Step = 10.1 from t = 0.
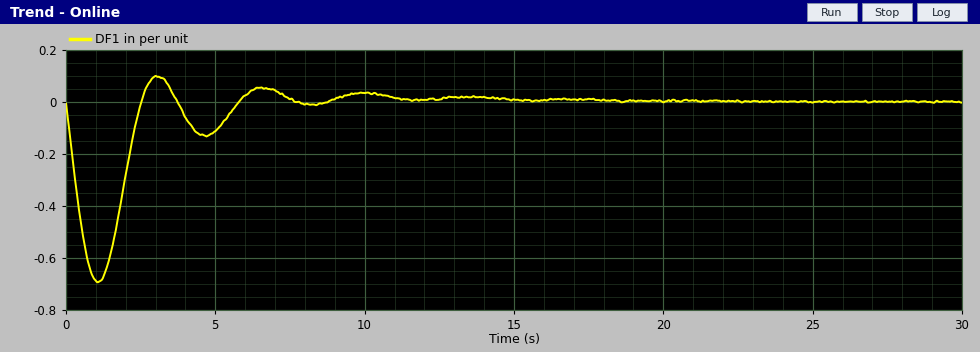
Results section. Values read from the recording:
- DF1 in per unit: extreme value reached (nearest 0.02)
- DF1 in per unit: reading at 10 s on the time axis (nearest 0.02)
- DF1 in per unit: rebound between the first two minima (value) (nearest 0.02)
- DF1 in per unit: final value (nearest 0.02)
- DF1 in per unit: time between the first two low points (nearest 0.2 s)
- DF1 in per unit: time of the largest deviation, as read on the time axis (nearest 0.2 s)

-0.70
0.04
0.10
0.00
3.6 s
1.0 s
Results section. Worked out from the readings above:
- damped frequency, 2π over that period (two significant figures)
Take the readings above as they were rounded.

1.7 rad/s
